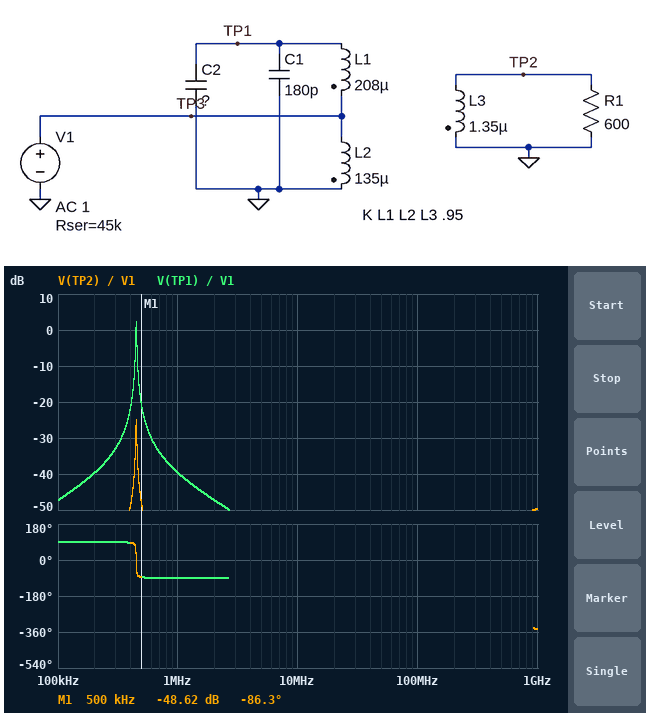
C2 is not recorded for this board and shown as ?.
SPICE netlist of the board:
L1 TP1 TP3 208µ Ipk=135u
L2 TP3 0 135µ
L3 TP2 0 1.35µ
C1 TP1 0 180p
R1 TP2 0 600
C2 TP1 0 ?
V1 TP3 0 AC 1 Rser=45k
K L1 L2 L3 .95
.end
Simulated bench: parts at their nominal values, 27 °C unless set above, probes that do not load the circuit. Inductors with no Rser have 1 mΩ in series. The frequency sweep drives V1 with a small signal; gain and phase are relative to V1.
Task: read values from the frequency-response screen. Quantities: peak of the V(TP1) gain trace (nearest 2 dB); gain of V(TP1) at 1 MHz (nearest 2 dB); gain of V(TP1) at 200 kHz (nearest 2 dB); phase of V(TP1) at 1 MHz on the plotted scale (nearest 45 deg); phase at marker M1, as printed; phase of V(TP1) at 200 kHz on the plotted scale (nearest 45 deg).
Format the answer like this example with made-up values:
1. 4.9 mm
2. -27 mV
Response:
1. 2 dB
2. -40 dB
3. -40 dB
4. -90 deg
5. -86.3 deg
6. 90 deg
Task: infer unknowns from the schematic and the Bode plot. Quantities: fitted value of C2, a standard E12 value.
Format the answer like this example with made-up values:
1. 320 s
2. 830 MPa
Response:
1. 10 pF
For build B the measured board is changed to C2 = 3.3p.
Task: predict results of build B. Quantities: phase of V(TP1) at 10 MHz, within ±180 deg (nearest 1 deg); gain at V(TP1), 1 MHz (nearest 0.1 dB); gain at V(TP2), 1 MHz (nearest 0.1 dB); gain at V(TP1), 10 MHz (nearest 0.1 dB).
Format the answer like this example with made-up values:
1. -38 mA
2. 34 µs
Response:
1. -90 deg
2. -39.3 dB
3. -66.6 dB
4. -61.3 dB
